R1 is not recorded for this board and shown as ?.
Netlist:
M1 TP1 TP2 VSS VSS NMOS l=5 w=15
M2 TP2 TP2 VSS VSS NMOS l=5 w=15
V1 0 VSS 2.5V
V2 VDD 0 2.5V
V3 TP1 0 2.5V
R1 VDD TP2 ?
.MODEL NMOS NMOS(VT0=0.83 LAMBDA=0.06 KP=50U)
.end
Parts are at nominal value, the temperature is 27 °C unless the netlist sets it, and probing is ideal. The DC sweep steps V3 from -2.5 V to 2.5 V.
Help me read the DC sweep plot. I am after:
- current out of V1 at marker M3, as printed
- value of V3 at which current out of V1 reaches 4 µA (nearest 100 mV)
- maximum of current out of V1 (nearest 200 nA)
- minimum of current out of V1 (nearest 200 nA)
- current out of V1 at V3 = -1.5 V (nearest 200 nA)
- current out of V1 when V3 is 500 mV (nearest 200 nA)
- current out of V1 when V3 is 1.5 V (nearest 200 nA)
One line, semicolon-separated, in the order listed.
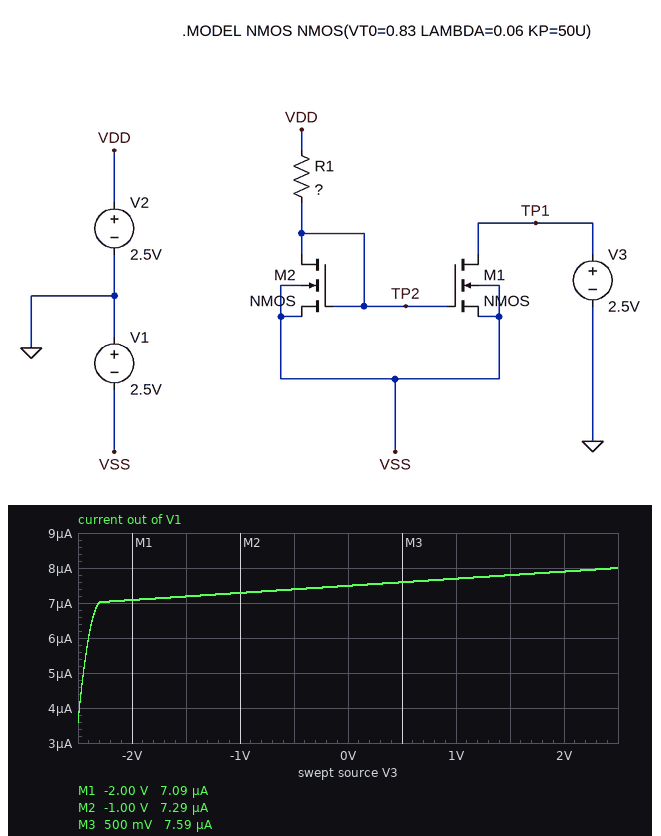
7.59 µA; -2.5 V; 8.0 µA; 3.6 µA; 7.2 µA; 7.6 µA; 7.8 µA
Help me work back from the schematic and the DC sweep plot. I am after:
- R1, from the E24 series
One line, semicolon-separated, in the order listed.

1.1 MΩ
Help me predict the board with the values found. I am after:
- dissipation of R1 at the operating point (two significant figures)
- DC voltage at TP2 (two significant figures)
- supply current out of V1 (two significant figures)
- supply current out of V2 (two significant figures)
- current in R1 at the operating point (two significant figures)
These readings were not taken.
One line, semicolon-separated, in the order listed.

14 µW; -1.5 V; 8.0 µA; 3.6 µA; 3.6 µA
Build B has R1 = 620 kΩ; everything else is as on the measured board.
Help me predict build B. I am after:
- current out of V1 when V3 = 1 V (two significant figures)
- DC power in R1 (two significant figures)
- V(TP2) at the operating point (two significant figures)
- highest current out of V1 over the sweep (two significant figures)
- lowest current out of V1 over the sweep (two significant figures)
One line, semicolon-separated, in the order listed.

13 µA; 24 µW; -1.4 V; 14 µA; 6.3 µA
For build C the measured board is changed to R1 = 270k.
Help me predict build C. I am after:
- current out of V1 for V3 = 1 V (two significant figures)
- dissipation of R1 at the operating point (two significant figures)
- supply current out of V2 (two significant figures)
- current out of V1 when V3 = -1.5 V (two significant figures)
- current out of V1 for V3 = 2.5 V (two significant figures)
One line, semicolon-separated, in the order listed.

30 µA; 52 µW; 14 µA; 28 µA; 31 µA
